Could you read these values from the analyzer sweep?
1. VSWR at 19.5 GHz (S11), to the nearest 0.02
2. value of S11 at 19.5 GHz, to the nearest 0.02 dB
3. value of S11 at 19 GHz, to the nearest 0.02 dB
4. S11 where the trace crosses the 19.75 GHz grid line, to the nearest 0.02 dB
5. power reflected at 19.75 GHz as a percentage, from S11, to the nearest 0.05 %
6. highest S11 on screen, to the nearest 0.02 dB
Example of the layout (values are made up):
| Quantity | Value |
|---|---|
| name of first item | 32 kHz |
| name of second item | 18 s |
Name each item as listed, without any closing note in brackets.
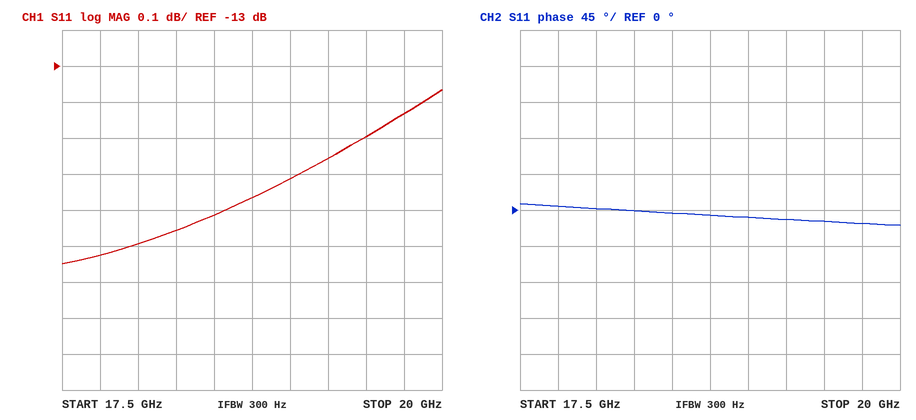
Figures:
| Quantity | Value |
|---|---|
| VSWR at 19.5 GHz (S11), to the nearest 0.02 | 1.56 |
| value of S11 at 19.5 GHz, to the nearest 0.02 dB | -13.20 dB |
| value of S11 at 19 GHz, to the nearest 0.02 dB | -13.32 dB |
| S11 where the trace crosses the 19.75 GHz grid line, to the nearest 0.02 dB | -13.14 dB |
| power reflected at 19.75 GHz as a percentage, from S11, to the nearest 0.05 % | 4.85 % |
| highest S11 on screen, to the nearest 0.02 dB | -13.06 dB |
